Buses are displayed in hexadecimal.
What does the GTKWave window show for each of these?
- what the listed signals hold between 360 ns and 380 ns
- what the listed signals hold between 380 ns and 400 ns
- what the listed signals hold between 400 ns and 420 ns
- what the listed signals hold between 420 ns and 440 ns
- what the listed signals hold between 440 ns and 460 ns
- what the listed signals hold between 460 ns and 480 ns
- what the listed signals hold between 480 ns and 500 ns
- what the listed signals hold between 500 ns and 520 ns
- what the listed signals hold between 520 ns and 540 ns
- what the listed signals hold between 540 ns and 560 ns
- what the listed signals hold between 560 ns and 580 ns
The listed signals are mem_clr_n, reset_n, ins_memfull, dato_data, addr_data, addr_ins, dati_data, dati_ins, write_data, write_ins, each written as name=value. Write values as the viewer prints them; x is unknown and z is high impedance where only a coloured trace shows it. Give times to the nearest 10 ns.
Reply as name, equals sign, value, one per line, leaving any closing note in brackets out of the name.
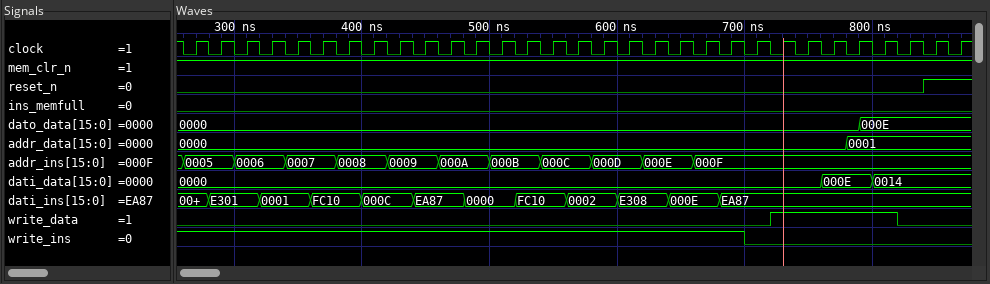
what the listed signals hold between 360 ns and 380 ns = mem_clr_n=1, reset_n=0, ins_memfull=0, dato_data=0000, addr_data=0000, addr_ins=0007, dati_data=0000, dati_ins=FC10, write_data=0, write_ins=1
what the listed signals hold between 380 ns and 400 ns = mem_clr_n=1, reset_n=0, ins_memfull=0, dato_data=0000, addr_data=0000, addr_ins=0008, dati_data=0000, dati_ins=FC10, write_data=0, write_ins=1
what the listed signals hold between 400 ns and 420 ns = mem_clr_n=1, reset_n=0, ins_memfull=0, dato_data=0000, addr_data=0000, addr_ins=0008, dati_data=0000, dati_ins=000C, write_data=0, write_ins=1
what the listed signals hold between 420 ns and 440 ns = mem_clr_n=1, reset_n=0, ins_memfull=0, dato_data=0000, addr_data=0000, addr_ins=0009, dati_data=0000, dati_ins=000C, write_data=0, write_ins=1
what the listed signals hold between 440 ns and 460 ns = mem_clr_n=1, reset_n=0, ins_memfull=0, dato_data=0000, addr_data=0000, addr_ins=0009, dati_data=0000, dati_ins=EA87, write_data=0, write_ins=1
what the listed signals hold between 460 ns and 480 ns = mem_clr_n=1, reset_n=0, ins_memfull=0, dato_data=0000, addr_data=0000, addr_ins=000A, dati_data=0000, dati_ins=EA87, write_data=0, write_ins=1
what the listed signals hold between 480 ns and 500 ns = mem_clr_n=1, reset_n=0, ins_memfull=0, dato_data=0000, addr_data=0000, addr_ins=000A, dati_data=0000, dati_ins=0000, write_data=0, write_ins=1
what the listed signals hold between 500 ns and 520 ns = mem_clr_n=1, reset_n=0, ins_memfull=0, dato_data=0000, addr_data=0000, addr_ins=000B, dati_data=0000, dati_ins=0000, write_data=0, write_ins=1
what the listed signals hold between 520 ns and 540 ns = mem_clr_n=1, reset_n=0, ins_memfull=0, dato_data=0000, addr_data=0000, addr_ins=000B, dati_data=0000, dati_ins=FC10, write_data=0, write_ins=1
what the listed signals hold between 540 ns and 560 ns = mem_clr_n=1, reset_n=0, ins_memfull=0, dato_data=0000, addr_data=0000, addr_ins=000C, dati_data=0000, dati_ins=FC10, write_data=0, write_ins=1
what the listed signals hold between 560 ns and 580 ns = mem_clr_n=1, reset_n=0, ins_memfull=0, dato_data=0000, addr_data=0000, addr_ins=000C, dati_data=0000, dati_ins=0002, write_data=0, write_ins=1
